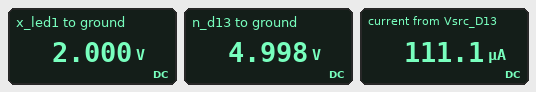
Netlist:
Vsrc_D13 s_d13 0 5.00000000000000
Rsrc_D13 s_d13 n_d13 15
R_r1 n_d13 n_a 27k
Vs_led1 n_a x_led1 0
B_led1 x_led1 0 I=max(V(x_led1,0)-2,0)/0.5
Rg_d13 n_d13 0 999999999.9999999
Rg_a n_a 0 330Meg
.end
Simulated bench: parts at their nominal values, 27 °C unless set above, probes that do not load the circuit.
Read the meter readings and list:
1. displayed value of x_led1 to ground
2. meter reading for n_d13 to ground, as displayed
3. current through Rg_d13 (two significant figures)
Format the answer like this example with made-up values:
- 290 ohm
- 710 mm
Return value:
- 2.000 V
- 4.998 V
- 5.0 nA
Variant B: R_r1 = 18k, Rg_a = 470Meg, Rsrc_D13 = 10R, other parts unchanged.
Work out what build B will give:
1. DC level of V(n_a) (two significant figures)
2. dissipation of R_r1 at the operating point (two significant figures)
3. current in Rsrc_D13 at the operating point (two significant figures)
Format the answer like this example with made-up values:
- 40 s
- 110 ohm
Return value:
- 2.0 V
- 500 µW
- 170 µA
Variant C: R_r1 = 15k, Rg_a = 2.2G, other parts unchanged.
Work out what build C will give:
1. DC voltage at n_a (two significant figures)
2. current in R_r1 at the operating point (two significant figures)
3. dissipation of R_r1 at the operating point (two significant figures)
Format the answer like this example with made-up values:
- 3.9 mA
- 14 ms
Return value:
- 2.0 V
- 200 µA
- 600 µW
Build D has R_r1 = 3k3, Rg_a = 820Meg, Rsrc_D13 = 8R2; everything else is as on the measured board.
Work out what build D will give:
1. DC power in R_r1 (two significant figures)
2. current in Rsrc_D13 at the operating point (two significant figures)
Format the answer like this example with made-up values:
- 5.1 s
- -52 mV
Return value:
- 2.7 mW
- 910 µA
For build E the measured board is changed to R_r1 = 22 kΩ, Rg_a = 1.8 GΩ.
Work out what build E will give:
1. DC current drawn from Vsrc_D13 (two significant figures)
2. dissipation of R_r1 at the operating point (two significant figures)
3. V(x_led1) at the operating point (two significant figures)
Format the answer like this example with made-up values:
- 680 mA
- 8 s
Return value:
- 140 µA
- 410 µW
- 2.0 V
